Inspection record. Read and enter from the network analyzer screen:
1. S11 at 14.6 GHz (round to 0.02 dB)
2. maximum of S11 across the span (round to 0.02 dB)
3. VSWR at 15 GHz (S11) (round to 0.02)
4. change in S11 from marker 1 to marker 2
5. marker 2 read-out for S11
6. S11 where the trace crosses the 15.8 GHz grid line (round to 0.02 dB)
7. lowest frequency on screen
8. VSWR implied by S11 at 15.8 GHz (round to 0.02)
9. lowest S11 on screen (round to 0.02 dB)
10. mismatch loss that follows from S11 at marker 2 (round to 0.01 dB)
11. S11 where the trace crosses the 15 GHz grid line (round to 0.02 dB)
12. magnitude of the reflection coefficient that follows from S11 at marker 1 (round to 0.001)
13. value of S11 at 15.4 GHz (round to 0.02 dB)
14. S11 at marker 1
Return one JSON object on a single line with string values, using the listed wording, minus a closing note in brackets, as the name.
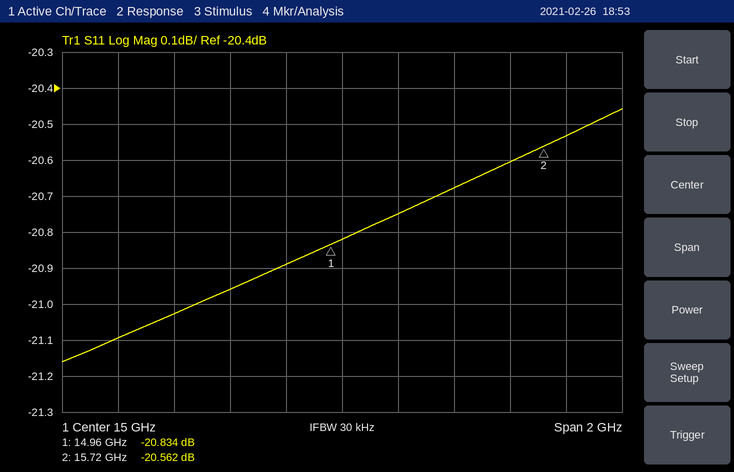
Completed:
{"S11 at 14.6 GHz": "-20.96 dB", "maximum of S11 across the span": "-20.46 dB", "VSWR at 15 GHz (S11)": "1.20", "change in S11 from marker 1 to marker 2": "0.272 dB", "marker 2 read-out for S11": "-20.562 dB", "S11 where the trace crosses the 15.8 GHz grid line": "-20.54 dB", "lowest frequency on screen": "14 GHz", "VSWR implied by S11 at 15.8 GHz": "1.20", "lowest S11 on screen": "-21.16 dB", "mismatch loss that follows from S11 at marker 2": "0.04 dB", "S11 where the trace crosses the 15 GHz grid line": "-20.82 dB", "magnitude of the reflection coefficient that follows from S11 at marker 1": "0.091", "value of S11 at 15.4 GHz": "-20.68 dB", "S11 at marker 1": "-20.834 dB"}
